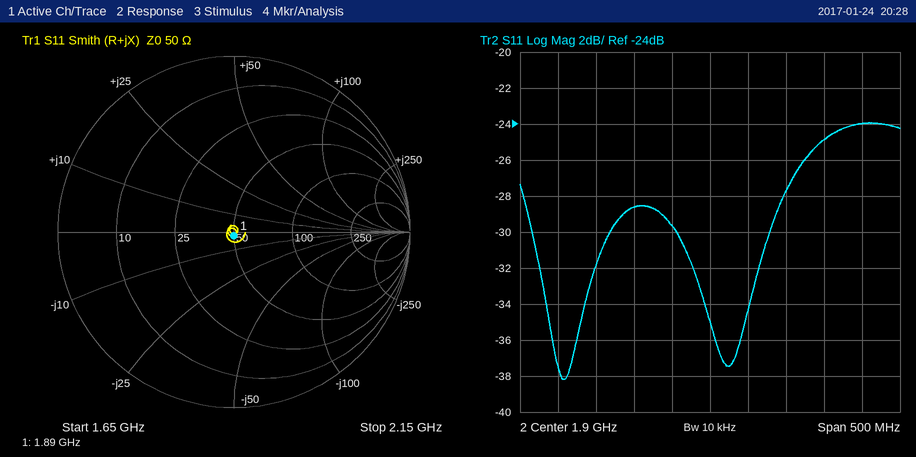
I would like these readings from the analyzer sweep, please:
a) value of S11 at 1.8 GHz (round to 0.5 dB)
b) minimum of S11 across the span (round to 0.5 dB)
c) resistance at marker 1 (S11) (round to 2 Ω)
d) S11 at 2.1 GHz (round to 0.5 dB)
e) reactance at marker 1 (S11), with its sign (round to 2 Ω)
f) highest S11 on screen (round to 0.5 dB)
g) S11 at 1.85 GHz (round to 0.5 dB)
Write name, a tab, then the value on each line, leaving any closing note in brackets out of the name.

value of S11 at 1.8 GHz	-28.5 dB
minimum of S11 across the span	-38.0 dB
resistance at marker 1 (S11)	50 Ω
S11 at 2.1 GHz	-24.0 dB
reactance at marker 1 (S11), with its sign	-2 Ω
highest S11 on screen	-24.0 dB
S11 at 1.85 GHz	-29.5 dB
